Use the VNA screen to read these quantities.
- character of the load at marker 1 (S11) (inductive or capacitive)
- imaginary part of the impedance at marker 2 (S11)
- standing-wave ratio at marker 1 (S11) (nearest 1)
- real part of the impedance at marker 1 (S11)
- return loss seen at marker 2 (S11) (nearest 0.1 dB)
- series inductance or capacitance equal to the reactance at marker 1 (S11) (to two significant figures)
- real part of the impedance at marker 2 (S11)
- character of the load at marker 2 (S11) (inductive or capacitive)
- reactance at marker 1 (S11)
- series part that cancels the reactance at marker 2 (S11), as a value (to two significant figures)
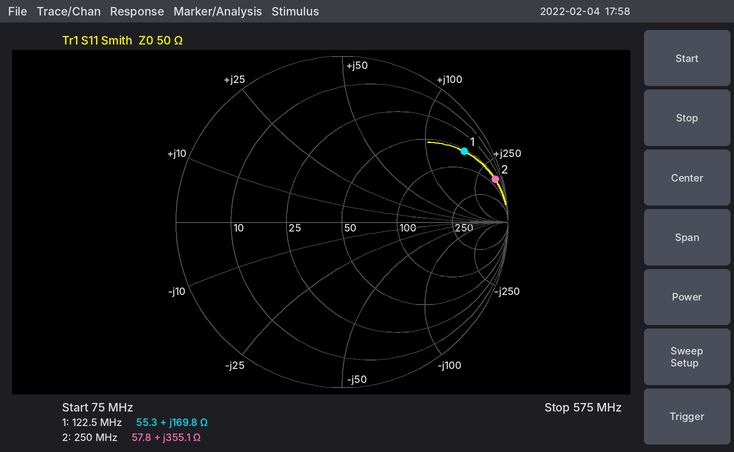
inductive
+355.1 Ω
12
55.3 Ω
0.4 dB
220 nH
57.8 Ω
inductive
+169.8 Ω
1.8 pF
